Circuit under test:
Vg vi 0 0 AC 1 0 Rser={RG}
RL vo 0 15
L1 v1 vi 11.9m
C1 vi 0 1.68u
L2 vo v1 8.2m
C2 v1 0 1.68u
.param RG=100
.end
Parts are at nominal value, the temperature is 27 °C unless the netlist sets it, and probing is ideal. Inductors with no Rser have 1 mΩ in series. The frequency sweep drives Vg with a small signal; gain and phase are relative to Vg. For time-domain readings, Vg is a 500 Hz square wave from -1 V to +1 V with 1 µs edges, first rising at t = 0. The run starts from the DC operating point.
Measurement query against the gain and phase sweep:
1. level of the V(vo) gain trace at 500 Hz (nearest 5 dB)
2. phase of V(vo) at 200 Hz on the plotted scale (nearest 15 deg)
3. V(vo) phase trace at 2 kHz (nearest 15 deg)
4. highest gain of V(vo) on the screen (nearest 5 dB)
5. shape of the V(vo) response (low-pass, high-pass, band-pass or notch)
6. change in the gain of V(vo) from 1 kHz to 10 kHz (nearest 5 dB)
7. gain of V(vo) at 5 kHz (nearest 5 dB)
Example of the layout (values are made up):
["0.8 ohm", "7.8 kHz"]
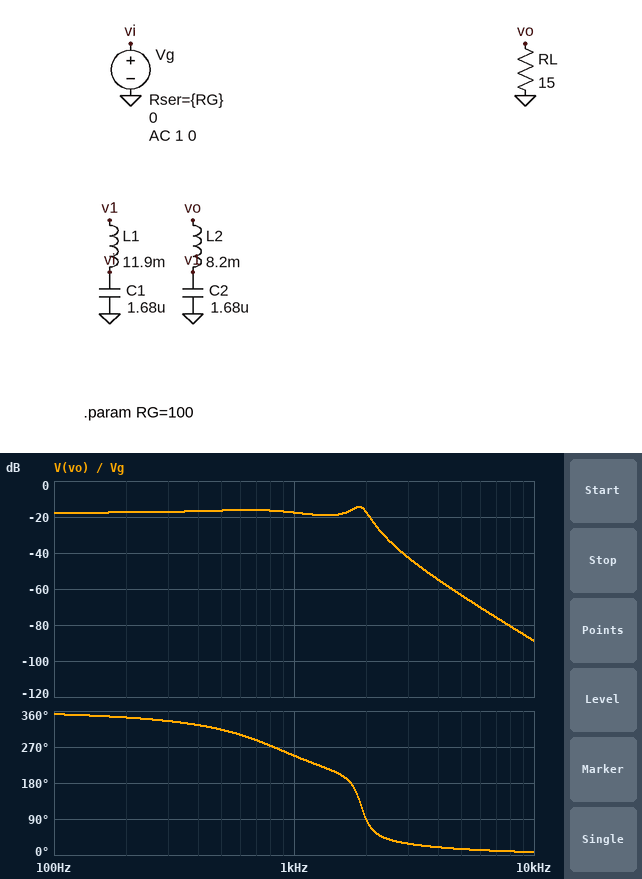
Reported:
["-15 dB", "345 deg", "90 deg", "-15 dB", "low-pass", "-70 dB", "-65 dB"]
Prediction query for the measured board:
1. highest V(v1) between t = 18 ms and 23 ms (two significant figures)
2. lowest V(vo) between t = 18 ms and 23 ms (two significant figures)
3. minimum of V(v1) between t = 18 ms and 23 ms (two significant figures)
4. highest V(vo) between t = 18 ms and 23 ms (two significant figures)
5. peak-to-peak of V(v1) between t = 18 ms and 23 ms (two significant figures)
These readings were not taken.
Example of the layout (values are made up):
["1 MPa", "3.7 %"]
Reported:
["660 mV", "-180 mV", "-660 mV", "180 mV", "1.3 V"]
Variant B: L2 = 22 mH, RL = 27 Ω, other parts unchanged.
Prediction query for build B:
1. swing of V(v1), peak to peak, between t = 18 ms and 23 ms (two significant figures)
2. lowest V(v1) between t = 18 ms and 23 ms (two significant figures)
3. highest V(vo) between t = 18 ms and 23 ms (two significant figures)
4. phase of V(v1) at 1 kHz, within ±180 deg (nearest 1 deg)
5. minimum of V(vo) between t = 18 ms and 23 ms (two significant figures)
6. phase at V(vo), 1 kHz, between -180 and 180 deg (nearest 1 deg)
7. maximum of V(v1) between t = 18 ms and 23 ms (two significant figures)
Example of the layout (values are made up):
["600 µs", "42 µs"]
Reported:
["2.4 V", "-1.2 V", "270 mV", "-58 deg", "-270 mV", "-137 deg", "1.2 V"]
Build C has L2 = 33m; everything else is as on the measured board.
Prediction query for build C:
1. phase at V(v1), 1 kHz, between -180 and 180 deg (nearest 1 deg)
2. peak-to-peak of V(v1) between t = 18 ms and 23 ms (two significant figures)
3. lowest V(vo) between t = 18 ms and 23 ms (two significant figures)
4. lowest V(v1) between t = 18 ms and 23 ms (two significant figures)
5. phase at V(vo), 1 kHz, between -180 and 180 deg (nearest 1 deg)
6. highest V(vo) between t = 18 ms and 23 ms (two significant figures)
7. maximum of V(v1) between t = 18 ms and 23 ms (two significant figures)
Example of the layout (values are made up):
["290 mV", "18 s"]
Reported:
["-64 deg", "2.9 V", "-150 mV", "-1.5 V", "-150 deg", "150 mV", "1.5 V"]
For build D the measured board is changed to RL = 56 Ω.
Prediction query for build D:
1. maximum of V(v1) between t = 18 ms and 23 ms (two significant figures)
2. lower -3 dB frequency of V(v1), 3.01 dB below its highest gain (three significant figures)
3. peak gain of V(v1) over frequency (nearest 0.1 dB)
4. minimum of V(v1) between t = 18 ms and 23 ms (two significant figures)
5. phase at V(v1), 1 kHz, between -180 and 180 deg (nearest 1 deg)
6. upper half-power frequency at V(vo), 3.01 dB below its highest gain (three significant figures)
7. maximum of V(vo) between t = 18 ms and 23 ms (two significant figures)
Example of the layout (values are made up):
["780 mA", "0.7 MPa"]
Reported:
["640 mV", "1.06 kHz", "-3.4 dB", "-640 mV", "-59 deg", "1.97 kHz", "460 mV"]
